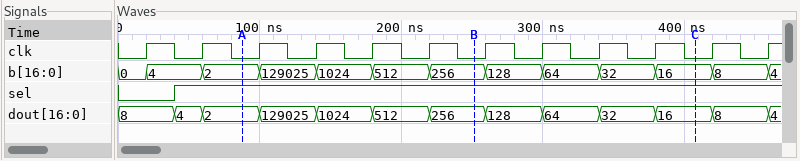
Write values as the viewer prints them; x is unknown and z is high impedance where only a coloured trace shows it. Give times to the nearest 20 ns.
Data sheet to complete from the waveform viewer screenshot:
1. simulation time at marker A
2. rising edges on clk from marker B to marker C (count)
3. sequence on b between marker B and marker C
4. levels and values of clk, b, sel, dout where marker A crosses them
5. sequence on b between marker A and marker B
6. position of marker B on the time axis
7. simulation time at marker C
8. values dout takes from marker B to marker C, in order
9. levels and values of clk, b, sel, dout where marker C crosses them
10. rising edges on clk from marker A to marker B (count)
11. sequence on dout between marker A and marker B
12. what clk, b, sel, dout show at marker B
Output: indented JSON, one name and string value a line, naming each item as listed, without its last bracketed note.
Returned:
{
  "simulation time at marker A": "80 ns",
  "rising edges on clk from marker B to marker C": "4",
  "sequence on b between marker B and marker C": "256, 128, 64, 32, 16",
  "levels and values of clk, b, sel, dout where marker A crosses them": "clk=0, b=2, sel=1, dout=2",
  "sequence on b between marker A and marker B": "2, 129025, 1024, 512, 256",
  "position of marker B on the time axis": "260 ns",
  "simulation time at marker C": "400 ns",
  "values dout takes from marker B to marker C, in order": "256, 128, 64, 32, 16",
  "levels and values of clk, b, sel, dout where marker C crosses them": "clk=0, b=16, sel=1, dout=16",
  "rising edges on clk from marker A to marker B": "4",
  "sequence on dout between marker A and marker B": "2, 129025, 1024, 512, 256",
  "what clk, b, sel, dout show at marker B": "clk=0, b=256, sel=1, dout=256"
}
